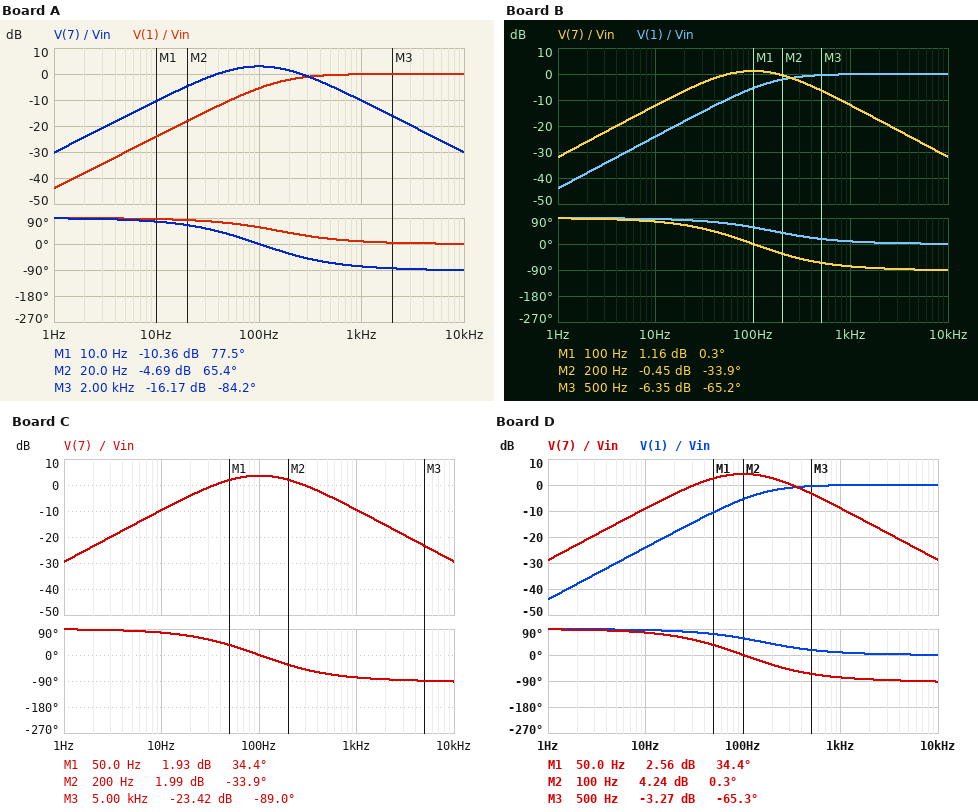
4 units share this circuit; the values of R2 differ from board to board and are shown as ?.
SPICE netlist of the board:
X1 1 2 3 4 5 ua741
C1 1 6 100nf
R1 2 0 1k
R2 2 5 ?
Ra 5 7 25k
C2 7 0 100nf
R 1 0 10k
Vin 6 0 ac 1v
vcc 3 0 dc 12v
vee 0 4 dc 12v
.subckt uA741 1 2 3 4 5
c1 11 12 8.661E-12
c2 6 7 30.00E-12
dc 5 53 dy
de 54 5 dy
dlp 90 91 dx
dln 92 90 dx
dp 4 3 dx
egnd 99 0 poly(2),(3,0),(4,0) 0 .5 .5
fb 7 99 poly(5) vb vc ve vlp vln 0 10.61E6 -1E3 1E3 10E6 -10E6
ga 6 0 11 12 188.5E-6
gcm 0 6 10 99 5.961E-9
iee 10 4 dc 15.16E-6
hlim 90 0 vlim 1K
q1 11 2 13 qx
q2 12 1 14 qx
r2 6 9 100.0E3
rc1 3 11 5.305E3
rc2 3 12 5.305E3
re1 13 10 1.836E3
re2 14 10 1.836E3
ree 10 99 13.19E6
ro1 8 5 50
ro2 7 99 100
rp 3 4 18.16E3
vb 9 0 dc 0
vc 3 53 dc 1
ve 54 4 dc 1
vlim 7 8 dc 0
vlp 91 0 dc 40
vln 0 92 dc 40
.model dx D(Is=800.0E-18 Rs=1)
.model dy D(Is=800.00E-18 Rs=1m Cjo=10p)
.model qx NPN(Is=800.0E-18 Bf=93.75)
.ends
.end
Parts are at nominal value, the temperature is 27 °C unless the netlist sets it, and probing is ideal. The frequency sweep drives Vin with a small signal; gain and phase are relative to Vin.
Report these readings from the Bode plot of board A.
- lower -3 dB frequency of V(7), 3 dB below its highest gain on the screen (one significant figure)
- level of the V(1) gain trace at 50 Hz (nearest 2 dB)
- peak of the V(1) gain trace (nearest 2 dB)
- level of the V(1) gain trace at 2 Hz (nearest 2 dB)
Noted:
40 Hz
-10 dB
0 dB
-38 dB
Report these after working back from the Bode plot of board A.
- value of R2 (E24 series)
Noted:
3.9 kΩ
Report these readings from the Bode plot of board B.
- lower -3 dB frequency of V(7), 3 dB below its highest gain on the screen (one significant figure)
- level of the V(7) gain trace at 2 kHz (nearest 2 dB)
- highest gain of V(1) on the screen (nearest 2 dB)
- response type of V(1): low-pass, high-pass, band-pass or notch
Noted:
40 Hz
-18 dB
0 dB
high-pass
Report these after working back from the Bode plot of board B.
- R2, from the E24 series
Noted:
3 kΩ
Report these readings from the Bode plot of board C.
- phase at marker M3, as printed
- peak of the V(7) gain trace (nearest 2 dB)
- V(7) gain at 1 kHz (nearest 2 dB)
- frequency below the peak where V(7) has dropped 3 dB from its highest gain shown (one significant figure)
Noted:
-89.0 deg
4 dB
-10 dB
40 Hz
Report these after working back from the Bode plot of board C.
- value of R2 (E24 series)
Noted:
4.3 kΩ
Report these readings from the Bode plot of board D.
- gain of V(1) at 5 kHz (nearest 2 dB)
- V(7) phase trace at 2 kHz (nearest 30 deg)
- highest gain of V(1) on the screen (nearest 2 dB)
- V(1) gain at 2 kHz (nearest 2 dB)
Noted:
0 dB
-90 deg
0 dB
0 dB
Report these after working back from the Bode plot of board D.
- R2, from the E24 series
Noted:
4.7 kΩ
